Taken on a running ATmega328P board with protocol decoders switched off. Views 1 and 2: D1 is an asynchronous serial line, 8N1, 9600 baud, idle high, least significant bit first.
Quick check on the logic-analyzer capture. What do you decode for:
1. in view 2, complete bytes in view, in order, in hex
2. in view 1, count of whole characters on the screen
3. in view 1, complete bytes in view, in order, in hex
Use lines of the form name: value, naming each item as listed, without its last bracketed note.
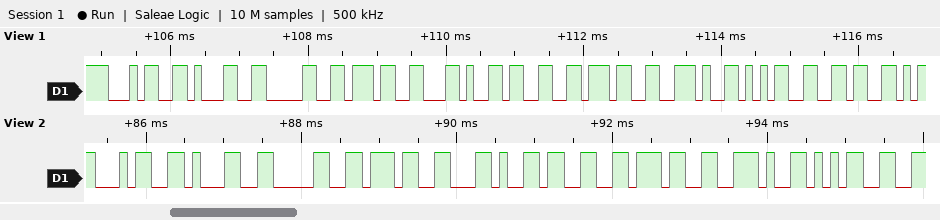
in view 2, complete bytes in view, in order, in hex: 0x34 0x31 0x30 0x37 0x2C 0x33 0x37 0x2E 0x35
in view 1, count of whole characters on the screen: 10
in view 1, complete bytes in view, in order, in hex: 34 31 30 37 2C 33 37 2E 35 36
